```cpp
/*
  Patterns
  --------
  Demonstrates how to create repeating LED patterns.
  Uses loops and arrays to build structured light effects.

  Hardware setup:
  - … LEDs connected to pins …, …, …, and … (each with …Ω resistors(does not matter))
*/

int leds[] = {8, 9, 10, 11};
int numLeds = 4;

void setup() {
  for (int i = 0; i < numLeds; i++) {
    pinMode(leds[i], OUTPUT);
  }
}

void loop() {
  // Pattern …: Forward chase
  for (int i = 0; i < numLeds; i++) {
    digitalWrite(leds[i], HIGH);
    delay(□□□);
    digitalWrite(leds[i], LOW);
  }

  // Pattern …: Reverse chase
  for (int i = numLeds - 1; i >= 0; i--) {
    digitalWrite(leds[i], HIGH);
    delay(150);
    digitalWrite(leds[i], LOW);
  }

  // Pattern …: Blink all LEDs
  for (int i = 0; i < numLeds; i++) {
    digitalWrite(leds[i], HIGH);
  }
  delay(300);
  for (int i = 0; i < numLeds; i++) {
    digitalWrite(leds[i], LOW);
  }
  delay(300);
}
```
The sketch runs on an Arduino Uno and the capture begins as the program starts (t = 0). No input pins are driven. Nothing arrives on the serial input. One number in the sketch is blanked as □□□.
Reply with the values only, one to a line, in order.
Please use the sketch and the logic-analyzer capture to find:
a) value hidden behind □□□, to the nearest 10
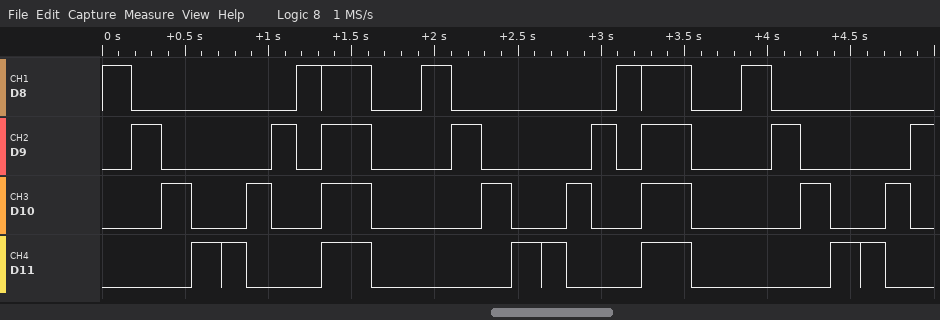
180
